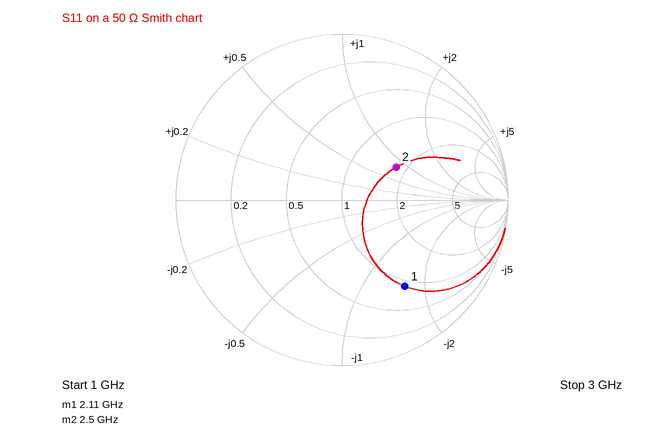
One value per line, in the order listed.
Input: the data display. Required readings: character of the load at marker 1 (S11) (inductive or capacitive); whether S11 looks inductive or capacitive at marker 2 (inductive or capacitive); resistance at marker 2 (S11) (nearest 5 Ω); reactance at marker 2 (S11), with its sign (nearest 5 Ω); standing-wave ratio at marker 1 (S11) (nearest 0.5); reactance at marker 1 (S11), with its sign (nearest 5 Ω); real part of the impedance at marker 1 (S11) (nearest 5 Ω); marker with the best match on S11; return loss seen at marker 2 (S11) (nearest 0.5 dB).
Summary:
capacitive
inductive
85 Ω
+40 Ω
4.5
-80 Ω
45 Ω
marker 2
8.5 dB
